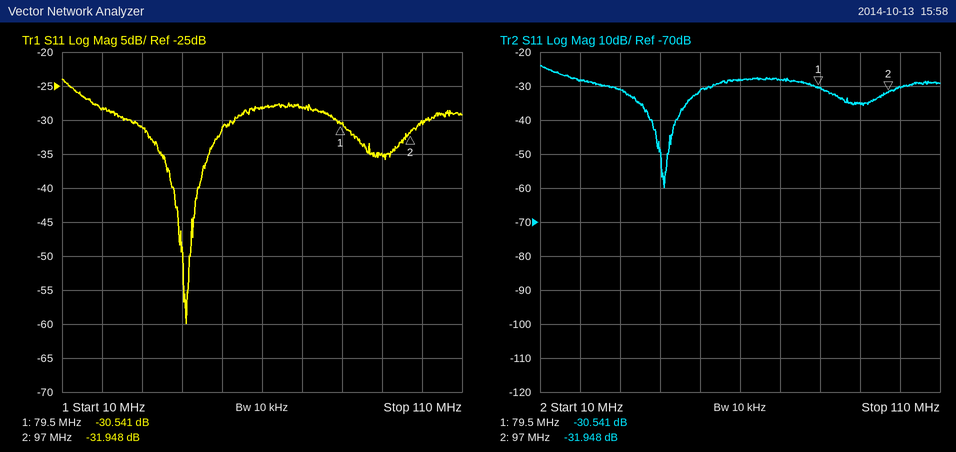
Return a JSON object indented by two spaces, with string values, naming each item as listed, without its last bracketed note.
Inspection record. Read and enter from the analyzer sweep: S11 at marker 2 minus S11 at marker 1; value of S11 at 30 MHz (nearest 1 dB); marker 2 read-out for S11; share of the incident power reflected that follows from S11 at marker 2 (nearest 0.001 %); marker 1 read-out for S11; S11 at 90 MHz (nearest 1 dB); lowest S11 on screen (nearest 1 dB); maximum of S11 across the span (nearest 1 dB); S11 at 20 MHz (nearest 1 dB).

{
  "S11 at marker 2 minus S11 at marker 1": "-1.407 dB",
  "value of S11 at 30 MHz": "-31 dB",
  "marker 2 read-out for S11": "-31.948 dB",
  "share of the incident power reflected that follows from S11 at marker 2": "0.064 %",
  "marker 1 read-out for S11": "-30.541 dB",
  "S11 at 90 MHz": "-35 dB",
  "lowest S11 on screen": "-60 dB",
  "maximum of S11 across the span": "-24 dB",
  "S11 at 20 MHz": "-28 dB"
}
